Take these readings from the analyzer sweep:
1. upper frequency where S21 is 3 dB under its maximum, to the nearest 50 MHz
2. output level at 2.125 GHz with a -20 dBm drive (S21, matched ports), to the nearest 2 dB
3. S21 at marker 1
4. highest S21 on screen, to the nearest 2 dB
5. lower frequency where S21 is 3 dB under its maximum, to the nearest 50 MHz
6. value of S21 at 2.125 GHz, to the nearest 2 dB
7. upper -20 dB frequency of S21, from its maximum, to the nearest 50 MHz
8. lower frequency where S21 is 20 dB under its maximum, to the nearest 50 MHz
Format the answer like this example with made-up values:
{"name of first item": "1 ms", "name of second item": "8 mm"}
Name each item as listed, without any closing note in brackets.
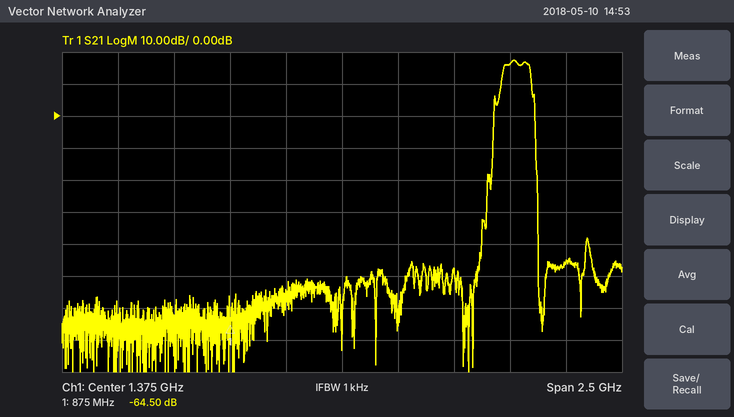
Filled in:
{"upper frequency where S21 is 3 dB under its maximum, to the nearest 50 MHz": "2.20 GHz", "output level at 2.125 GHz with a -20 dBm drive (S21, matched ports), to the nearest 2 dB": "-4 dBm", "S21 at marker 1": "-64.50 dB", "highest S21 on screen, to the nearest 2 dB": "18 dB", "lower frequency where S21 is 3 dB under its maximum, to the nearest 50 MHz": "2.10 GHz", "value of S21 at 2.125 GHz, to the nearest 2 dB": "16 dB", "upper -20 dB frequency of S21, from its maximum, to the nearest 50 MHz": "2.25 GHz", "lower frequency where S21 is 20 dB under its maximum, to the nearest 50 MHz": "2.05 GHz"}
